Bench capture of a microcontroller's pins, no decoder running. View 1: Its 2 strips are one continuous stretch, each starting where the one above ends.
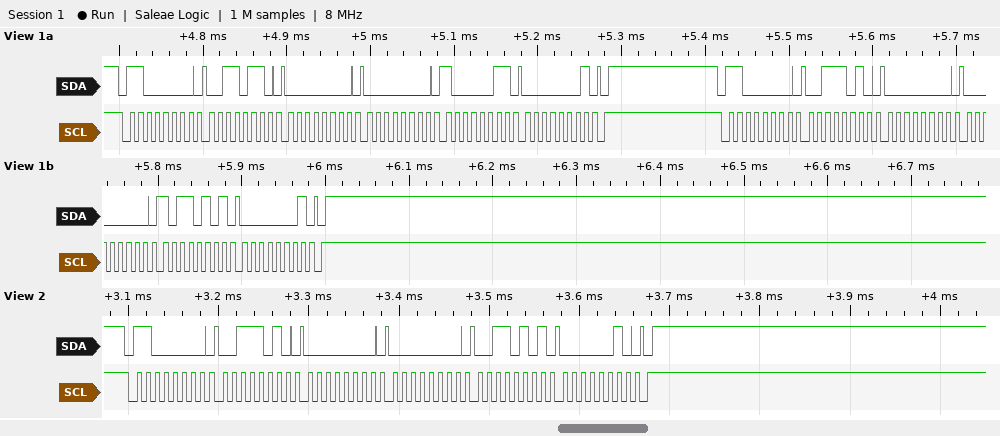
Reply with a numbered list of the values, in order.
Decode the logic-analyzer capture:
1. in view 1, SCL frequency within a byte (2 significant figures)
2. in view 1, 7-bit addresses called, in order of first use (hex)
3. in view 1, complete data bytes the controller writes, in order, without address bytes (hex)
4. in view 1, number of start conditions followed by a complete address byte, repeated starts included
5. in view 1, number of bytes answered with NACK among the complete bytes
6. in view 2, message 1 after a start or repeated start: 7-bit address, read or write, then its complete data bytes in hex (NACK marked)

1. 100 kHz
2. 0x60
3. 36 00 00 83 01 3A 00 00 B5 01
4. 2
5. 0
6. 0x60 write: 3A 00 00 35 02
